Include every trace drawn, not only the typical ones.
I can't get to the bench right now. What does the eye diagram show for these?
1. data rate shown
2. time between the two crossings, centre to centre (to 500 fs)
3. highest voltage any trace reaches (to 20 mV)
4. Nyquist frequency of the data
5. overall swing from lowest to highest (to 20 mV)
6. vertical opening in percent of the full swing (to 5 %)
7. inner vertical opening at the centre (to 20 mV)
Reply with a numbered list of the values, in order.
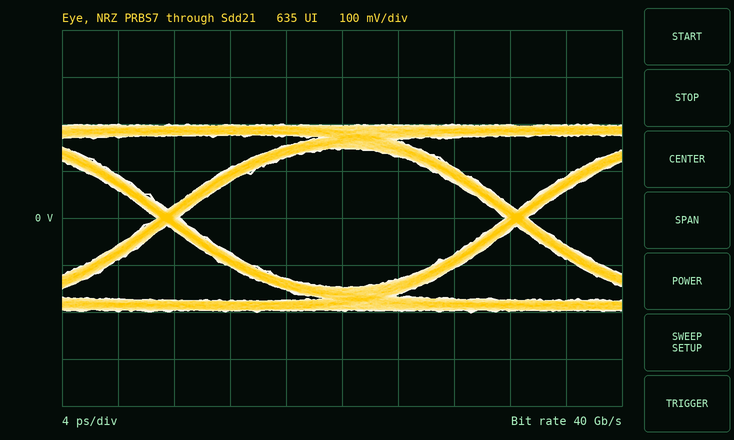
1. 40 Gb/s
2. 25.0 ps
3. 200 mV
4. 20 GHz
5. 400 mV
6. 75 %
7. 300 mV
